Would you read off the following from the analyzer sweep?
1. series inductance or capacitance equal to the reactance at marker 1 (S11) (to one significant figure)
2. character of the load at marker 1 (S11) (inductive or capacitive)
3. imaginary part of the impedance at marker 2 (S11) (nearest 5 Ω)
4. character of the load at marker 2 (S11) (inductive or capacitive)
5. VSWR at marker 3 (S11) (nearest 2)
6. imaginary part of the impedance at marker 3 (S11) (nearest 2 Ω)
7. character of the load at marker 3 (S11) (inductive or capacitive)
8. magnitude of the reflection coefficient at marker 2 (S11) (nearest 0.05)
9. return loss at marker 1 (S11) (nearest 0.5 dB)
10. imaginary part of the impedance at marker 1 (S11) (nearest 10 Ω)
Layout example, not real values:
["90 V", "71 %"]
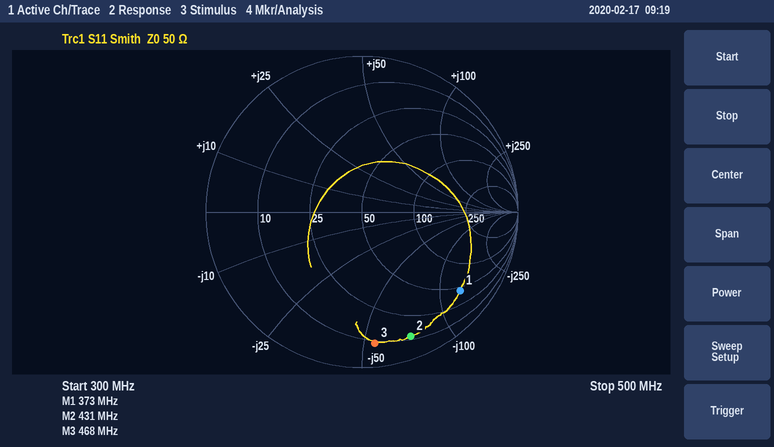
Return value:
["3 pF", "capacitive", "-70 Ω", "capacitive", "12", "-54 Ω", "capacitive", "0.85", "2.0 dB", "-130 Ω"]
